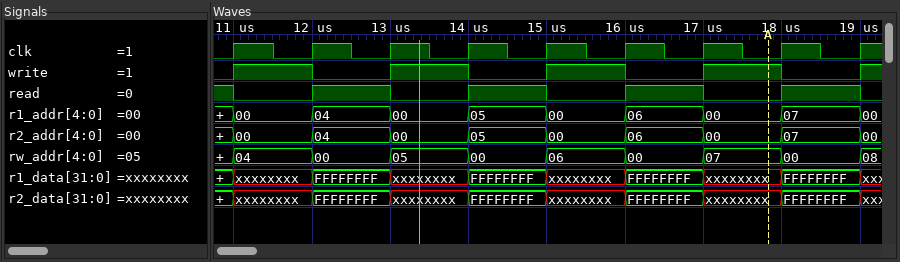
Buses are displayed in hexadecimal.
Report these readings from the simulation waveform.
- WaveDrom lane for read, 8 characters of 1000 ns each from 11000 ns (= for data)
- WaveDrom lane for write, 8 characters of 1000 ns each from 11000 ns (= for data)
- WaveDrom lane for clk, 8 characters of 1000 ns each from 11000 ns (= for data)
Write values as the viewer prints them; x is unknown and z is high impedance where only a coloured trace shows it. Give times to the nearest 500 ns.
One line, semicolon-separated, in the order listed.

{name: 'read', wave: '01010101'}; {name: 'write', wave: '10101010'}; {name: 'clk', wave: 'p.......'}
